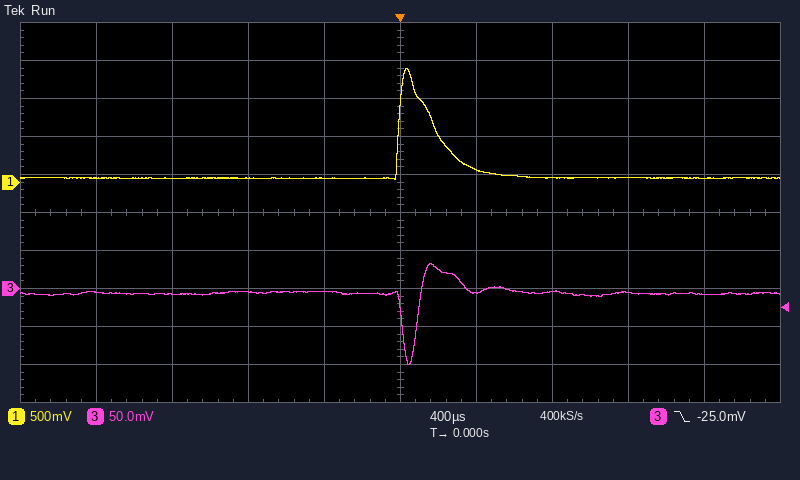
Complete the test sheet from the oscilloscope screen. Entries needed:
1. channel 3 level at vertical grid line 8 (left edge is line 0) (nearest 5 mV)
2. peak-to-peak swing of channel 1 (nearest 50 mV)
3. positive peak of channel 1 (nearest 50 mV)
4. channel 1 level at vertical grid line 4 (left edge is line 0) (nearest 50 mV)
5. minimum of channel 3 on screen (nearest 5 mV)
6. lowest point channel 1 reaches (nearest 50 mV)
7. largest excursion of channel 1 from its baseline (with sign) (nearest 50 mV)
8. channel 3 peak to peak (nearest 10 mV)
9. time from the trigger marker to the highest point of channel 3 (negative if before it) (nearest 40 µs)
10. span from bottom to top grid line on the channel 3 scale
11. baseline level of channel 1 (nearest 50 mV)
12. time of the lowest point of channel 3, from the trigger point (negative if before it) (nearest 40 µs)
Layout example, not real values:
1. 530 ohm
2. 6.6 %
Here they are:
1. -5 mV
2. 1.45 V
3. 1.50 V
4. 50 mV
5. -100 mV
6. 50 mV
7. +1.45 V
8. 130 mV
9. +160 µs
10. 500 mV
11. 50 mV
12. +40 µs
